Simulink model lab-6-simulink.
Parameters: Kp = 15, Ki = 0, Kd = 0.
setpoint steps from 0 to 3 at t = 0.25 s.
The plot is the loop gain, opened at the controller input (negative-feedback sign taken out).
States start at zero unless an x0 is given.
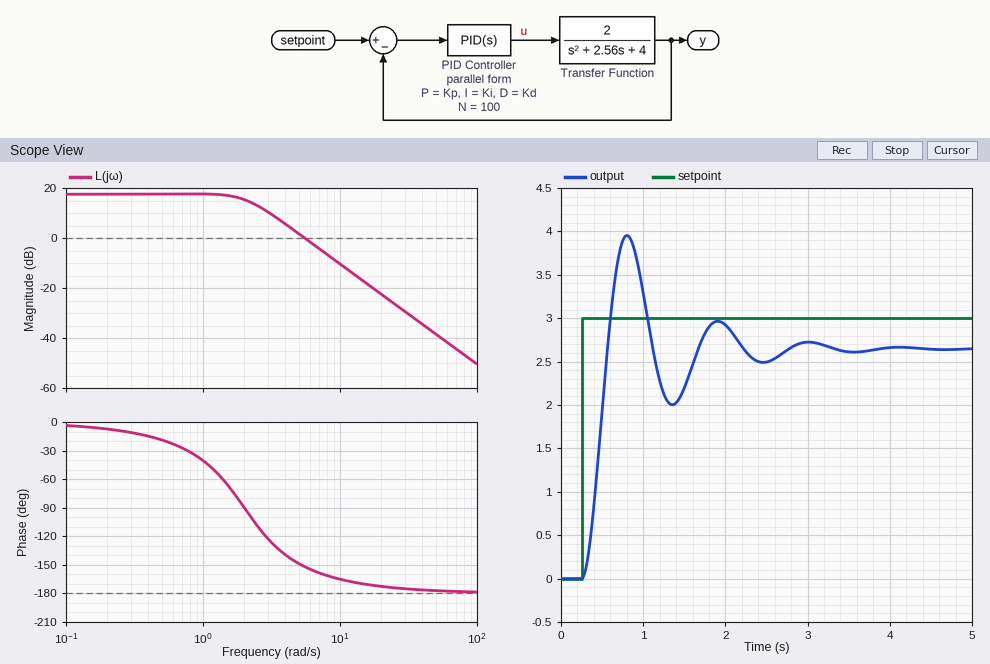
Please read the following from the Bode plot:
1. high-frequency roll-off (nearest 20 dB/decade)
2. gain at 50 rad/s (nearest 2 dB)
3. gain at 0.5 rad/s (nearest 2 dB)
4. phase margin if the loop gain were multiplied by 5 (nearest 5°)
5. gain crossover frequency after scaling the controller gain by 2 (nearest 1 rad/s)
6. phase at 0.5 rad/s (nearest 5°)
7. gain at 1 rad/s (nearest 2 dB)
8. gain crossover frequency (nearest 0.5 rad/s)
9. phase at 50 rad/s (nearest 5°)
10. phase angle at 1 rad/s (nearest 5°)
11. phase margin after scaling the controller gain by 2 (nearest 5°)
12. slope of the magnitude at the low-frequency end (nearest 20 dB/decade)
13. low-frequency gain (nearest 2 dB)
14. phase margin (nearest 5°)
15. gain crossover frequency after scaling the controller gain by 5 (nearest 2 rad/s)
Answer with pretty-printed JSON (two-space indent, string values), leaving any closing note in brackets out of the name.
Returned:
{
  "high-frequency roll-off": "-40 dB/decade",
  "gain at 50 rad/s": "-38 dB",
  "gain at 0.5 rad/s": "18 dB",
  "phase margin if the loop gain were multiplied by 5": "10°",
  "gain crossover frequency after scaling the controller gain by 2": "8 rad/s",
  "phase at 0.5 rad/s": "-20°",
  "gain at 1 rad/s": "18 dB",
  "gain crossover frequency": "5.5 rad/s",
  "phase at 50 rad/s": "-175°",
  "phase angle at 1 rad/s": "-40°",
  "phase margin after scaling the controller gain by 2": "20°",
  "slope of the magnitude at the low-frequency end": "0 dB/decade",
  "low-frequency gain": "18 dB",
  "phase margin": "30°",
  "gain crossover frequency after scaling the controller gain by 5": "12 rad/s"
}
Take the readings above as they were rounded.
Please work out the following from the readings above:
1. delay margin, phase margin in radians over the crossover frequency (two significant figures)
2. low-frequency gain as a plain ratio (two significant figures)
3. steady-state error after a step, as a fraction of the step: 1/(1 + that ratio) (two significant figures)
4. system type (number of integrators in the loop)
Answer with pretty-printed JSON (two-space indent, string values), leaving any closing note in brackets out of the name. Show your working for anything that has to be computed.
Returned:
{
  "delay margin, phase margin in radians over the crossover frequency": "30 × π / 180 / 5.5 = 0.095 s",
  "low-frequency gain as a plain ratio": "10^(18 / 20) = 7.9",
  "steady-state error after a step, as a fraction of the step: 1/(1 + that ratio)": "1 / (1 + 7.9) = 0.11",
  "system type": "0"
}
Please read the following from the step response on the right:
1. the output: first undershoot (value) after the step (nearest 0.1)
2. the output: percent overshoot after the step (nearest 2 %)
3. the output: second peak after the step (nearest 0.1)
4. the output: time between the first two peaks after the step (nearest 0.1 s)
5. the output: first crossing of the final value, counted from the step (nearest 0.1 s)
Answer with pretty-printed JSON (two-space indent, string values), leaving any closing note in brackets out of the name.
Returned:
{
  "the output: first undershoot (value) after the step": "2.0",
  "the output: percent overshoot after the step": "50 %",
  "the output: second peak after the step": "3.0",
  "the output: time between the first two peaks after the step": "1.1 s",
  "the output: first crossing of the final value, counted from the step": "0.3 s"
}
